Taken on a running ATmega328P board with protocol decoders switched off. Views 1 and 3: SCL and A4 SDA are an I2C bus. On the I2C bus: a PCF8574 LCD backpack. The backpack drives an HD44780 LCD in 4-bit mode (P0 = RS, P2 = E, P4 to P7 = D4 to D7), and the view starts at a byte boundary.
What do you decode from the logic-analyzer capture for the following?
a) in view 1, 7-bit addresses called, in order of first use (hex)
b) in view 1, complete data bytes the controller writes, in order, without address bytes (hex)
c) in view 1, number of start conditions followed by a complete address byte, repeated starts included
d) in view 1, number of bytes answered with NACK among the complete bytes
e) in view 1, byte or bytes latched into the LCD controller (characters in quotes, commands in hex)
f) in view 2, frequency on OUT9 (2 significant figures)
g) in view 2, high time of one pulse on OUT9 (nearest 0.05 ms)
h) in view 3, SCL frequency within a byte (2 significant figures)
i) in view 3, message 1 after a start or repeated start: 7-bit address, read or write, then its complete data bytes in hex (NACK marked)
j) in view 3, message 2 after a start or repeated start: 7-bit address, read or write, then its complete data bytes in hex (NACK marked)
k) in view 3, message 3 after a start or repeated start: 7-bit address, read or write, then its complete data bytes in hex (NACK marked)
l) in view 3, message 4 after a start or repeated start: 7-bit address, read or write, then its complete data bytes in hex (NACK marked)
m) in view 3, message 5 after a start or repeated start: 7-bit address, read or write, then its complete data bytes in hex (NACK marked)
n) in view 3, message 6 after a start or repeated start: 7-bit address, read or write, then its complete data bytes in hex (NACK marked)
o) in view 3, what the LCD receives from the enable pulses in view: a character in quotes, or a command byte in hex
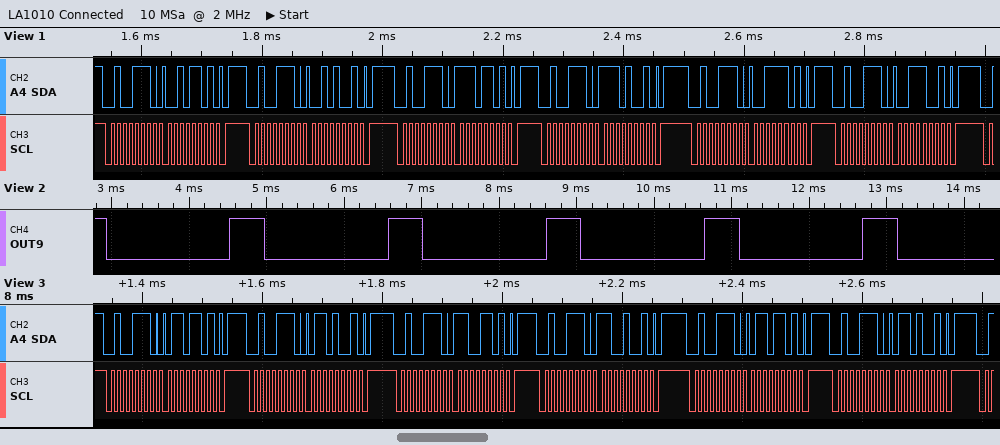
0x27
2D 29 ED E9 3D 39
6
0
'.'
490 Hz
0.45 ms
100 kHz
0x27 write: 6D
0x27 write: 69
0x27 write: CD
0x27 write: C9
0x27 write: 6D
0x27 write: 69
'l'
